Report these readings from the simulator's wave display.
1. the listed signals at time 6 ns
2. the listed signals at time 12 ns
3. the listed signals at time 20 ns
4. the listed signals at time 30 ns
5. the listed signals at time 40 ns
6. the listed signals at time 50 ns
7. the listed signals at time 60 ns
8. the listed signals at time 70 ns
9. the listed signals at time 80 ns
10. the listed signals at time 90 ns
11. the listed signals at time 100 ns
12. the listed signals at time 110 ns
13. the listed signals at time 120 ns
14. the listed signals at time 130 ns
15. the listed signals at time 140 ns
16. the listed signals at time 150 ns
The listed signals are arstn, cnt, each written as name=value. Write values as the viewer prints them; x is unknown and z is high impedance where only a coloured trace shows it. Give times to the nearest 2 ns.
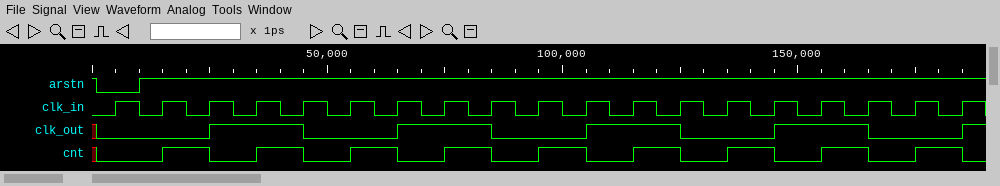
arstn=0, cnt=0
arstn=1, cnt=0
arstn=1, cnt=1
arstn=1, cnt=0
arstn=1, cnt=1
arstn=1, cnt=0
arstn=1, cnt=1
arstn=1, cnt=0
arstn=1, cnt=1
arstn=1, cnt=0
arstn=1, cnt=1
arstn=1, cnt=0
arstn=1, cnt=1
arstn=1, cnt=0
arstn=1, cnt=1
arstn=1, cnt=0
